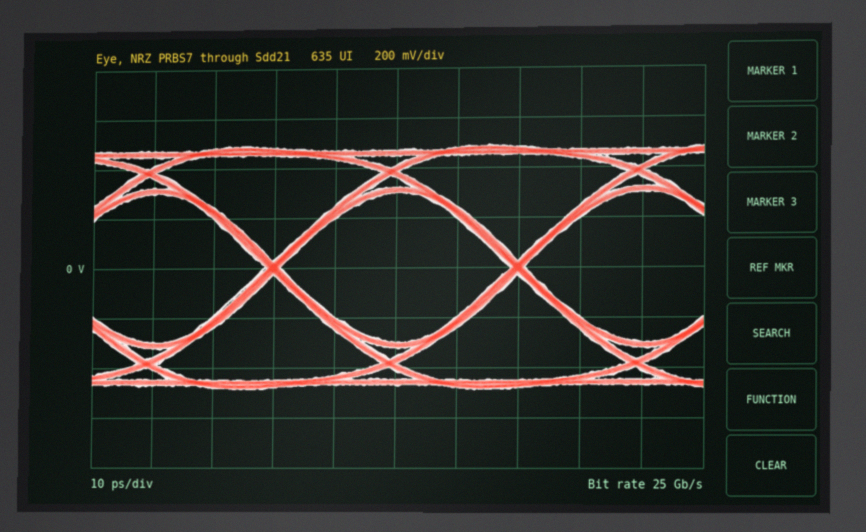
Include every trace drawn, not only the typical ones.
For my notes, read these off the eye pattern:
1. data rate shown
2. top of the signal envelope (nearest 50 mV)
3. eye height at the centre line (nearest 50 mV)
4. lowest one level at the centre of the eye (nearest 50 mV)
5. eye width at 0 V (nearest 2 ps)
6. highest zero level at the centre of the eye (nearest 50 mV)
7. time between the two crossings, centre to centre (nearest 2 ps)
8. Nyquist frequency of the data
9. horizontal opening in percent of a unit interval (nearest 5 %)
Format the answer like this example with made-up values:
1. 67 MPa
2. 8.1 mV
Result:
1. 25 Gb/s
2. 500 mV
3. 600 mV
4. 300 mV
5. 38 ps
6. -300 mV
7. 40 ps
8. 12.5 GHz
9. 95 %
